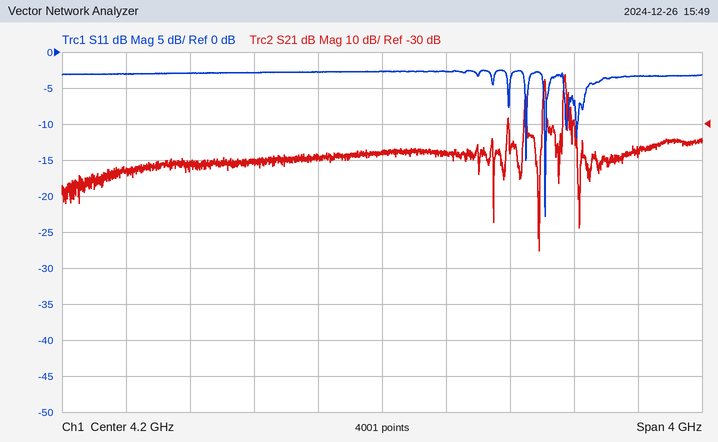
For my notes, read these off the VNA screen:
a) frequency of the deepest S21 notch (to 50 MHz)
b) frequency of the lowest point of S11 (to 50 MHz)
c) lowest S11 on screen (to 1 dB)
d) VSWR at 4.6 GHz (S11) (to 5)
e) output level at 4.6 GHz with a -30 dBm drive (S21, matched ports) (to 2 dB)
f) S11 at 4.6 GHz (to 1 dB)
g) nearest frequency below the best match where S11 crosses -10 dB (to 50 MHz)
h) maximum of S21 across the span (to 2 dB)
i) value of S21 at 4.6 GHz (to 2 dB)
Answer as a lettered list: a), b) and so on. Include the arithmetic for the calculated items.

a) 5.20 GHz
b) 5.20 GHz
c) -23 dB
d) |Γ| = 10^(-3/20) = 0.7079; VSWR = (1 + 0.7079)/(1 − 0.7079) ≈ 5.85, so 5 to the nearest 5
e) -30 dBm + (-38 dB) = -68 dBm
f) -3 dB
g) 5.20 GHz
h) -16 dB
i) -38 dB
